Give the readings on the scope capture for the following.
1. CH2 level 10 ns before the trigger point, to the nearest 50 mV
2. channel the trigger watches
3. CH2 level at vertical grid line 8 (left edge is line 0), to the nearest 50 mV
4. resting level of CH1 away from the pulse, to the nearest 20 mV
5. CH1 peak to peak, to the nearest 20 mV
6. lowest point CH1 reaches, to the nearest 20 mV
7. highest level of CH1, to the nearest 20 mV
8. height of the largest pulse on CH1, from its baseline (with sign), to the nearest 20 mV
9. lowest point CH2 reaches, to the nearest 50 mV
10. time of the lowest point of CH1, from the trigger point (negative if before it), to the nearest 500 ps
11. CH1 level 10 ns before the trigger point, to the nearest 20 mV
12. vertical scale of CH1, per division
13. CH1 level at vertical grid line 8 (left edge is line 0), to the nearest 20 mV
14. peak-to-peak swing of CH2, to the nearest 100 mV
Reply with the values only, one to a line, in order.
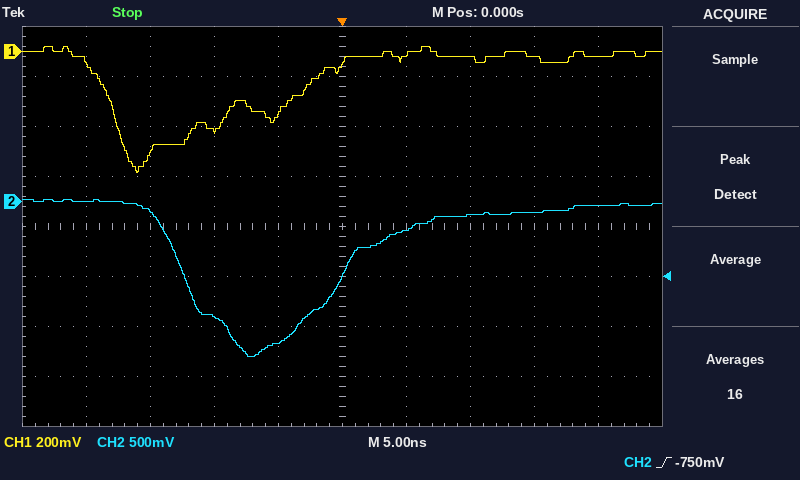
-1.15 V
CH2
-100 mV
-20 mV
500 mV
-480 mV
20 mV
-460 mV
-1.55 V
-16.0 ns
-320 mV
200 mV
-20 mV
1.60 V
